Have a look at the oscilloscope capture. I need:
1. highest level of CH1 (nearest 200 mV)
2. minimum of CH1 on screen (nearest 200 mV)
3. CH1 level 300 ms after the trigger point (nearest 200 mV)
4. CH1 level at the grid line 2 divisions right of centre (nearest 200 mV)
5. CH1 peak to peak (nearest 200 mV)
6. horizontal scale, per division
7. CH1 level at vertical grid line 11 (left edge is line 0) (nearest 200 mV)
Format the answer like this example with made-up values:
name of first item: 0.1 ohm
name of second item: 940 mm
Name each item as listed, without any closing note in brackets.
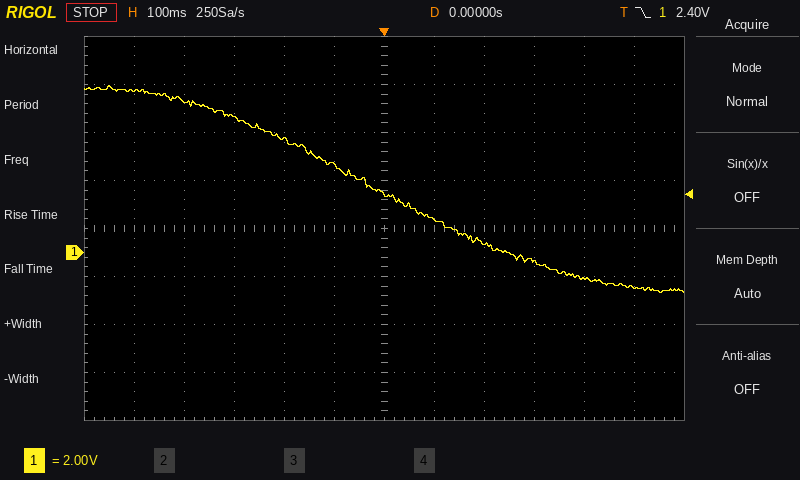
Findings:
highest level of CH1: 7.0 V
minimum of CH1 on screen: -1.6 V
CH1 level 300 ms after the trigger point: -400 mV
CH1 level at the grid line 2 divisions right of centre: 400 mV
CH1 peak to peak: 8.6 V
horizontal scale, per division: 100 ms
CH1 level at vertical grid line 11 (left edge is line 0): -1.4 V
